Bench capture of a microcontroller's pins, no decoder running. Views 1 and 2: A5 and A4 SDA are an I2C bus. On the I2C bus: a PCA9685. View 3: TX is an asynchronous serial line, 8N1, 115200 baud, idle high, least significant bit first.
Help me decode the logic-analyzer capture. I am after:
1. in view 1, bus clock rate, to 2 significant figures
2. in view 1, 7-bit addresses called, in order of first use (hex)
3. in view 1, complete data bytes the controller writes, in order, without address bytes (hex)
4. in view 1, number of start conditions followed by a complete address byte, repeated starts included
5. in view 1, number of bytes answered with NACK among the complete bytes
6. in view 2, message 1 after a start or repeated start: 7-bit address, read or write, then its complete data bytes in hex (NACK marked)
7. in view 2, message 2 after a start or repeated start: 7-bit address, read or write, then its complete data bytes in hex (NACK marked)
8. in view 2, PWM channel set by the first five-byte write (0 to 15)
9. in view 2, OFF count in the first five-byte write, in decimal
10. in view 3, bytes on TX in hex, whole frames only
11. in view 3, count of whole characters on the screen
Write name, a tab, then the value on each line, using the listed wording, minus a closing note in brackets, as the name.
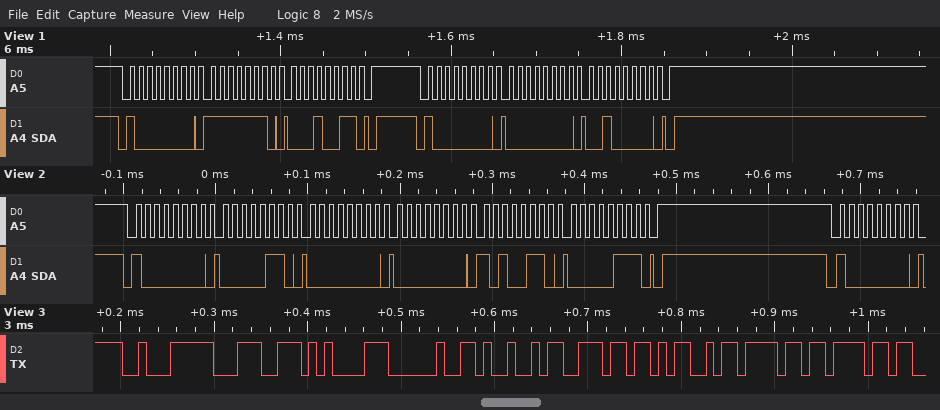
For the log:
in view 1, bus clock rate, to 2 significant figures	100 kHz
in view 1, 7-bit addresses called, in order of first use	0x40
in view 1, complete data bytes the controller writes, in order, without address bytes	FE 13 00 20
in view 1, number of start conditions followed by a complete address byte, repeated starts included	2
in view 1, number of bytes answered with NACK among the complete bytes	0
in view 2, message 1 after a start or repeated start: 7-bit address, read or write, then its complete data bytes in hex	0x40 write: 06 00 00 A6 07
in view 2, message 2 after a start or repeated start: 7-bit address, read or write, then its complete data bytes in hex	0x40 write
in view 2, PWM channel set by the first five-byte write	0
in view 2, OFF count in the first five-byte write, in decimal	1958
in view 3, bytes on TX in hex, whole frames only	E2 9C 85 20 49 6E 4D 6F 6F
in view 3, count of whole characters on the screen	9
